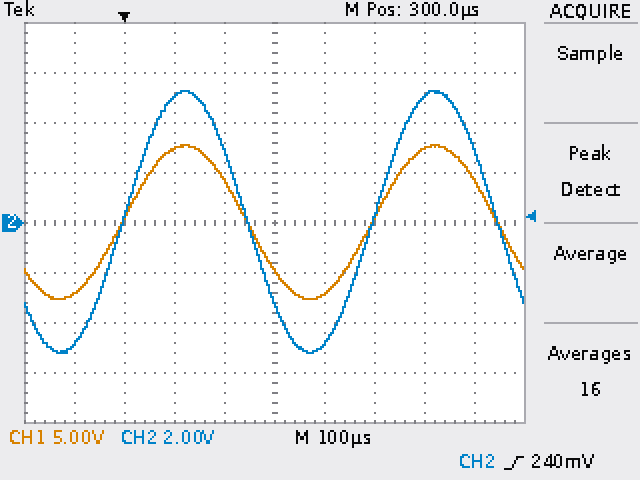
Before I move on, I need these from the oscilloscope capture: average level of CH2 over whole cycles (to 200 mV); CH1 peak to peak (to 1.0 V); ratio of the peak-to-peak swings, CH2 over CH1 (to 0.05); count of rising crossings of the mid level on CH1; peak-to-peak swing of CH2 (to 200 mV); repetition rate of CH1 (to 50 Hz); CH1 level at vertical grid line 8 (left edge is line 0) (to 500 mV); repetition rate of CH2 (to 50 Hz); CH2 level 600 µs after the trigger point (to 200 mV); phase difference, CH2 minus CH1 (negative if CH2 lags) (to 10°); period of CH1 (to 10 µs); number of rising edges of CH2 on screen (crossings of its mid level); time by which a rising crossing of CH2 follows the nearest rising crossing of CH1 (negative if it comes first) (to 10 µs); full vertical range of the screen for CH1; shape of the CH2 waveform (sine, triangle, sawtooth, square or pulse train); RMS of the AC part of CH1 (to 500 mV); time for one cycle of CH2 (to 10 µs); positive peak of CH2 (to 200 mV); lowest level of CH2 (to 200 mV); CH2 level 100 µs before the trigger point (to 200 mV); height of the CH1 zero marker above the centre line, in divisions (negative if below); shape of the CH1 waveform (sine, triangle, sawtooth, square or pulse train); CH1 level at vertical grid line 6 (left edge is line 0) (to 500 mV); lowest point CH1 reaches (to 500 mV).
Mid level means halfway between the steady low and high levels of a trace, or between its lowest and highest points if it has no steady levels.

0.0 V
15.0 V
0.70
2
10.4 V
2.00 kHz
7.5 V
2.00 kHz
5.0 V
0°
500 µs
2
0 µs
40 V
sine
5.5 V
500 µs
5.2 V
-5.2 V
-4.8 V
0.0 div
sine
-7.0 V
-7.5 V
